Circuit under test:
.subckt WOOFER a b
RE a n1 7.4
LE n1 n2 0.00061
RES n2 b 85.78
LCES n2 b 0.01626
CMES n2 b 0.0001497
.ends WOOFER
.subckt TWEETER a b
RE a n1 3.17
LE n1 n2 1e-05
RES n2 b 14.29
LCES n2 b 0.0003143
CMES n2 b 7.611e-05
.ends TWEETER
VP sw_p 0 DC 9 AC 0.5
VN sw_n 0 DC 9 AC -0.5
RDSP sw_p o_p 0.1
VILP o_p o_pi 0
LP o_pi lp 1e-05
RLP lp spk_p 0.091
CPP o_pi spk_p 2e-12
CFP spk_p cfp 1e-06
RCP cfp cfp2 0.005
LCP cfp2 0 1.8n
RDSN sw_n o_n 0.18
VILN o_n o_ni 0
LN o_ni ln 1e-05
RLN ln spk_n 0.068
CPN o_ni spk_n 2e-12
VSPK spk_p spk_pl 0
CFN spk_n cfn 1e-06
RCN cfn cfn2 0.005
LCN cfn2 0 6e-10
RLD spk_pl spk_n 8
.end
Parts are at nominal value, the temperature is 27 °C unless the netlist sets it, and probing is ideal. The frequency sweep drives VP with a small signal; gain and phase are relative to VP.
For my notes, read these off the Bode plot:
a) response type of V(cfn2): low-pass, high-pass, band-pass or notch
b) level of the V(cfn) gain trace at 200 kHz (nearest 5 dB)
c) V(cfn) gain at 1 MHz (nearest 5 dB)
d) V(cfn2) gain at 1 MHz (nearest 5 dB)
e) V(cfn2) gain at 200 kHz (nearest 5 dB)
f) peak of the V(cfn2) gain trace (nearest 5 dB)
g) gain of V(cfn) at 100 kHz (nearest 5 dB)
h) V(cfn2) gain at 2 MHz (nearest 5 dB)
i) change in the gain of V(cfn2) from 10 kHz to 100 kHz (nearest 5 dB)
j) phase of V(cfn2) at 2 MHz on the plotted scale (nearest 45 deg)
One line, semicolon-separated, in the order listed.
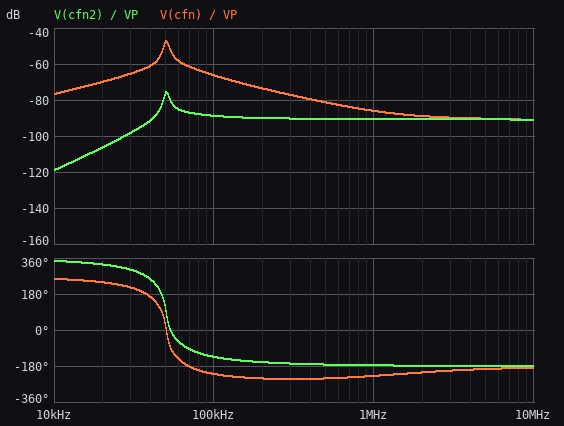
high-pass; -75 dB; -85 dB; -90 dB; -90 dB; -75 dB; -65 dB; -90 dB; 30 dB; -180 deg
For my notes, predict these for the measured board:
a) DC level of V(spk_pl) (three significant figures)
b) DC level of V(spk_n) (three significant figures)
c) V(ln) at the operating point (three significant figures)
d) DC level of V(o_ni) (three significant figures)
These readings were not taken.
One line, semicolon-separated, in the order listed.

9.00 V; 9.00 V; 9.00 V; 9.00 V
